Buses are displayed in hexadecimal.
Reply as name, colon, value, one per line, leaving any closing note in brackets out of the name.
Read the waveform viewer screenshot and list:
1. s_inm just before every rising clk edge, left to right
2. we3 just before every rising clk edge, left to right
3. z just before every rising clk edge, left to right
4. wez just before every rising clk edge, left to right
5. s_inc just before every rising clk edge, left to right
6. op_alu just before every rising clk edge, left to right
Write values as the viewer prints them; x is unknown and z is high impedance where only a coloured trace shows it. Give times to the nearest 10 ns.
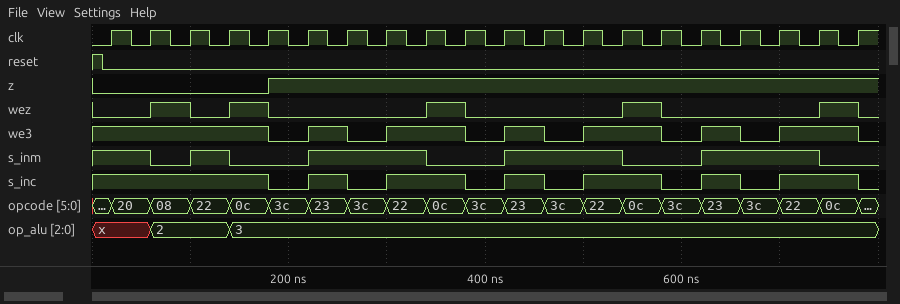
s_inm just before every rising clk edge, left to right: 1 1 0 1 0 0 1 1 1 0 0 1 1 1 0 0 1 1 1 0
we3 just before every rising clk edge, left to right: 1 1 1 1 1 0 1 0 1 1 0 1 0 1 1 0 1 0 1 1
z just before every rising clk edge, left to right: 0 0 0 0 0 1 1 1 1 1 1 1 1 1 1 1 1 1 1 1
wez just before every rising clk edge, left to right: 0 0 1 0 1 0 0 0 0 1 0 0 0 0 1 0 0 0 0 1
s_inc just before every rising clk edge, left to right: 1 1 1 1 1 0 1 0 1 1 0 1 0 1 1 0 1 0 1 1
op_alu just before every rising clk edge, left to right: x, x, 2, 2, 3, 3, 3, 3, 3, 3, 3, 3, 3, 3, 3, 3, 3, 3, 3, 3
